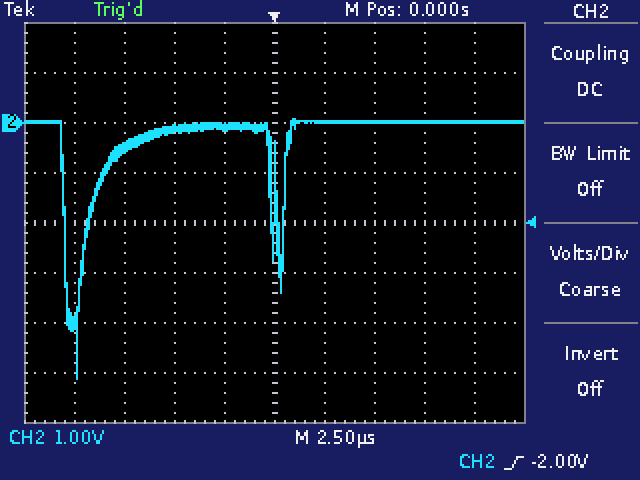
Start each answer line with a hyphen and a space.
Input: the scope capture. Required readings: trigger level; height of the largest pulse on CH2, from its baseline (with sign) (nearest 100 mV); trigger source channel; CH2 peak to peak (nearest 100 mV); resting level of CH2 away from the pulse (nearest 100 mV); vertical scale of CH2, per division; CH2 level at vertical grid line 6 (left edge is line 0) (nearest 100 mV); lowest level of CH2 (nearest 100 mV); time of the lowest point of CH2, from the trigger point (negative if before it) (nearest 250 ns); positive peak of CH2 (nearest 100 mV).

- -2.00 V
- -5.1 V
- CH2
- 5.2 V
- 0.0 V
- 1 V
- 0.0 V
- -5.1 V
- -9.75 µs
- 100 mV
